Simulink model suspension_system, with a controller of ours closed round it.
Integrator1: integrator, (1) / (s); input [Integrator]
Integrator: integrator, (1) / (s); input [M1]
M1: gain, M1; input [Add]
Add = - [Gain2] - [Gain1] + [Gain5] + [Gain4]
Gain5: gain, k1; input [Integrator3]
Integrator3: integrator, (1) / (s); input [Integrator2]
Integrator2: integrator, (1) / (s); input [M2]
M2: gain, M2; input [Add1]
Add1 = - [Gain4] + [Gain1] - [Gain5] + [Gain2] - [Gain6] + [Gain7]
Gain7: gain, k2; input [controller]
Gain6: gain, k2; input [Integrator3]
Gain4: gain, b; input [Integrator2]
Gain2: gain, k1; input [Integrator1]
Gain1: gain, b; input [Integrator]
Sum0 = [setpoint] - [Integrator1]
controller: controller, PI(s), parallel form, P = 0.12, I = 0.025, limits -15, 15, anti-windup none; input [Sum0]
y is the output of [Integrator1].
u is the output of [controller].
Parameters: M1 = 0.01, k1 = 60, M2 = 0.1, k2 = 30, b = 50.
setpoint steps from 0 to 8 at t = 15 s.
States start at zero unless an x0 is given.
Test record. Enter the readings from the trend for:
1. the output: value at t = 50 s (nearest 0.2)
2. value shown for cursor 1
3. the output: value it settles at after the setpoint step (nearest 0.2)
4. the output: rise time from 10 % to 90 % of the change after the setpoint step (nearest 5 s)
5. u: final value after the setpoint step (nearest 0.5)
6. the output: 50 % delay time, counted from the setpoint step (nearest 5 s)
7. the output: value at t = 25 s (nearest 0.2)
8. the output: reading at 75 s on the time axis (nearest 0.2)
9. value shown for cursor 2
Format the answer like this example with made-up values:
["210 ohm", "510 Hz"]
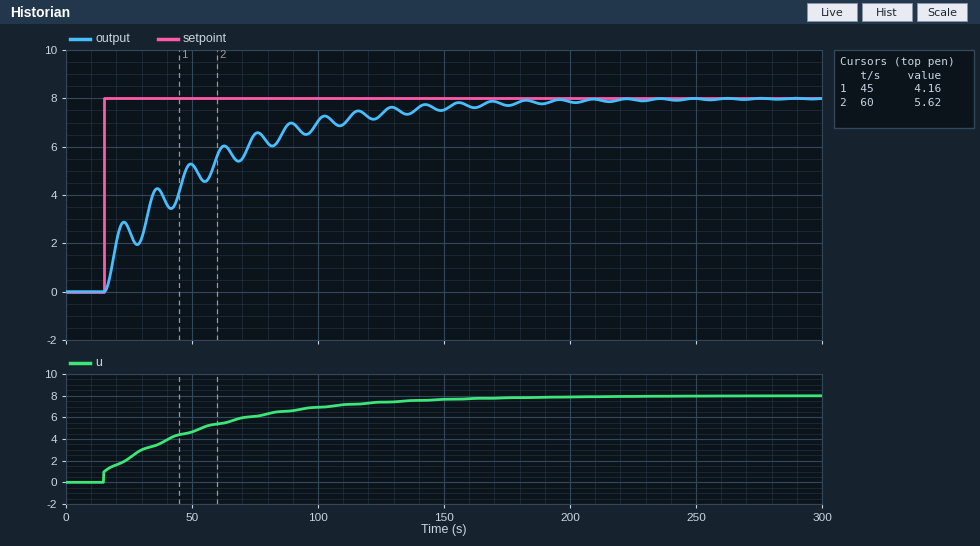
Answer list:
["5.2", "4.16", "8.0", "85 s", "8.0", "20 s", "2.6", "6.6", "5.62"]
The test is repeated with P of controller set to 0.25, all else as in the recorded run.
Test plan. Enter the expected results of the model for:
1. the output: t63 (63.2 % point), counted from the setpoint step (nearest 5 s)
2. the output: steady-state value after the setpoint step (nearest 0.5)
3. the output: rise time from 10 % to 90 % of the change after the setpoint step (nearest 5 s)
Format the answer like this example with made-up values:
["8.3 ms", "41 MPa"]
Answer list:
["30 s", "8.0", "90 s"]
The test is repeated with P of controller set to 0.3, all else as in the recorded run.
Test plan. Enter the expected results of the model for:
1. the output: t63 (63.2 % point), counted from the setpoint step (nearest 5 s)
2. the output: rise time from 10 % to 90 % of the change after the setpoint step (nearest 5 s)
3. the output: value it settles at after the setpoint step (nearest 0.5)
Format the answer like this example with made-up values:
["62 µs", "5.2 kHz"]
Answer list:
["20 s", "90 s", "8.0"]
